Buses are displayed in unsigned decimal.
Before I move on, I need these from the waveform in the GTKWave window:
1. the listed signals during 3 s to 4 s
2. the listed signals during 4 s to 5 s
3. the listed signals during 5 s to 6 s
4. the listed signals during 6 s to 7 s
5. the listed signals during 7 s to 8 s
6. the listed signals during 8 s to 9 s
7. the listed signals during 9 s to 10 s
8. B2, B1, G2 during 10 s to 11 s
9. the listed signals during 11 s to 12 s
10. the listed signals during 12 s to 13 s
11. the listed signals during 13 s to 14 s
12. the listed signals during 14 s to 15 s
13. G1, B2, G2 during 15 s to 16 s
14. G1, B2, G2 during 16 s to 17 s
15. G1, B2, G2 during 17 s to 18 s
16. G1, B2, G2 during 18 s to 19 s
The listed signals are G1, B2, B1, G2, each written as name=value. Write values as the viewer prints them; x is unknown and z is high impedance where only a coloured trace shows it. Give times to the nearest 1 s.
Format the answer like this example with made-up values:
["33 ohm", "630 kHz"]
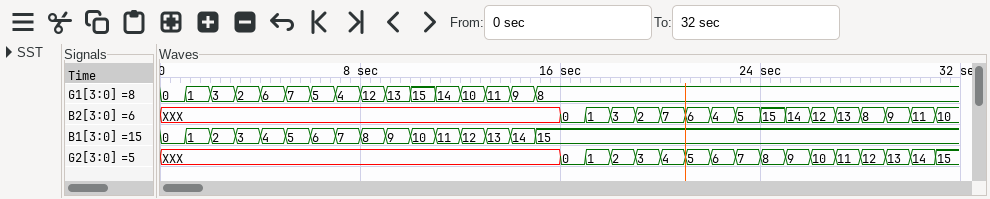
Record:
["G1=2, B2=XXX, B1=3, G2=XXX", "G1=6, B2=XXX, B1=4, G2=XXX", "G1=7, B2=XXX, B1=5, G2=XXX", "G1=5, B2=XXX, B1=6, G2=XXX", "G1=4, B2=XXX, B1=7, G2=XXX", "G1=12, B2=XXX, B1=8, G2=XXX", "G1=13, B2=XXX, B1=9, G2=XXX", "B2=XXX, B1=10, G2=XXX", "G1=14, B2=XXX, B1=11, G2=XXX", "G1=10, B2=XXX, B1=12, G2=XXX", "G1=11, B2=XXX, B1=13, G2=XXX", "G1=9, B2=XXX, B1=14, G2=XXX", "G1=8, B2=XXX, G2=XXX", "G1=8, B2=0, G2=0", "G1=8, B2=1, G2=1", "G1=8, B2=3, G2=2"]
